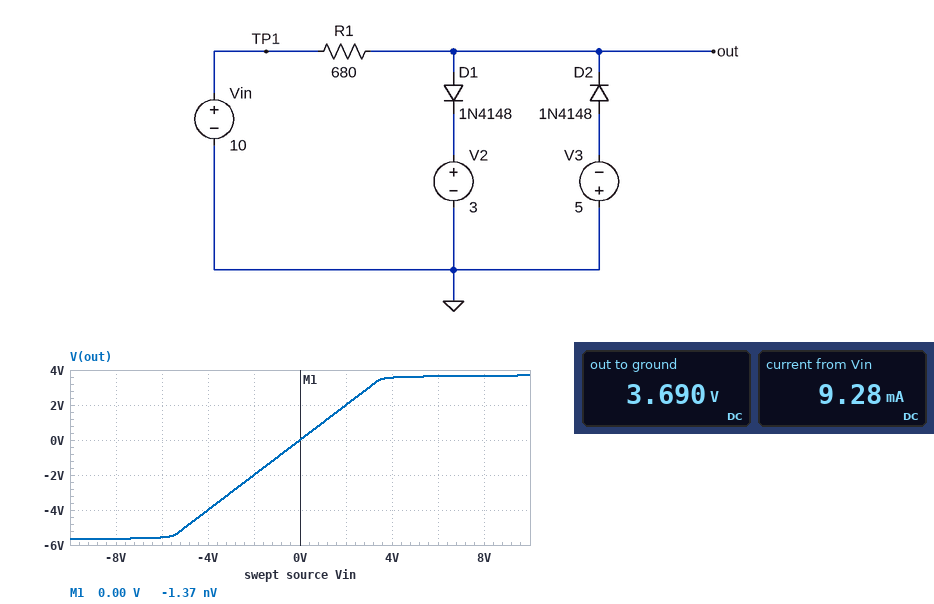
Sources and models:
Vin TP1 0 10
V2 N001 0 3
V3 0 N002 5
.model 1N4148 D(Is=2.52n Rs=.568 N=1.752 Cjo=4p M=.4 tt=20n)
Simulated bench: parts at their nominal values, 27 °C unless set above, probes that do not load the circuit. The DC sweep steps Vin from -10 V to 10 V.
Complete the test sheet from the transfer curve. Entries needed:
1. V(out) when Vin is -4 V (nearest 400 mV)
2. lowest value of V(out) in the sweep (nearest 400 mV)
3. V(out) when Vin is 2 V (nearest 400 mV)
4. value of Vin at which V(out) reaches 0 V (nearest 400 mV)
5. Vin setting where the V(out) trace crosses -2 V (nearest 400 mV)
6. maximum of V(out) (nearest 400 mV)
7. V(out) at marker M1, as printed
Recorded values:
-4.0 V
-5.6 V
2.0 V
0 V
-2.0 V
3.6 V
-1.37 nV
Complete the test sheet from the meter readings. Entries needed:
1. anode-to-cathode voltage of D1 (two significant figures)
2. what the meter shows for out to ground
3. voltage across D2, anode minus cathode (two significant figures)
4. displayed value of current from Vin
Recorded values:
690 mV
3.690 V
-8.7 V
9.28 mA
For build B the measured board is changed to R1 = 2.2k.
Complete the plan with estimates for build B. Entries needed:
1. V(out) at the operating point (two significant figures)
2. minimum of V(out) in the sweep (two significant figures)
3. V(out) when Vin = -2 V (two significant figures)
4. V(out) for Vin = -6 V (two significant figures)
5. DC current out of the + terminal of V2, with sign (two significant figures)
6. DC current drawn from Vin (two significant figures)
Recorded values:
3.6 V
-5.6 V
-2.0 V
-5.5 V
-2.9 mA
2.9 mA
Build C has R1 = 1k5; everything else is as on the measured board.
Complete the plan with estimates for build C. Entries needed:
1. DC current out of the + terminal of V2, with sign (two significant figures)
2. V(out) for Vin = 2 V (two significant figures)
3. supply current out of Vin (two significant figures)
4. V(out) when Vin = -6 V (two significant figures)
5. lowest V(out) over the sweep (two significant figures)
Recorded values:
-4.2 mA
2.0 V
4.2 mA
-5.5 V
-5.6 V
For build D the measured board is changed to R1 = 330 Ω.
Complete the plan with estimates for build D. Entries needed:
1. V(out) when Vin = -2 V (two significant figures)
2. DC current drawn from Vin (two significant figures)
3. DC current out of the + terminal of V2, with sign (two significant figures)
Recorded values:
-2.0 V
19 mA
-19 mA
